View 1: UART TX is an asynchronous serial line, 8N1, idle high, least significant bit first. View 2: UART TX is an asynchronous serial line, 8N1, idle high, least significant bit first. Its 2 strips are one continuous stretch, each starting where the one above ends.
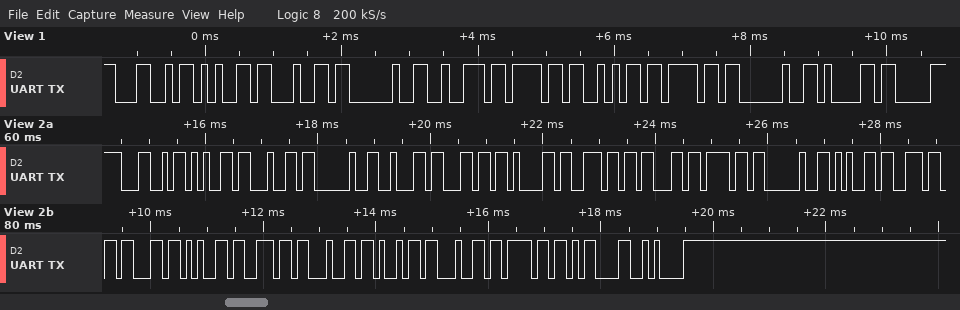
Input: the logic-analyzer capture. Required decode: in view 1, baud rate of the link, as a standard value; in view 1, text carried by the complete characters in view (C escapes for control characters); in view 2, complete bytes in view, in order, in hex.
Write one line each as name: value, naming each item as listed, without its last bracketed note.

in view 1, baud rate of the link, as a standard value: 9600 baud
in view 1, text carried by the complete characters in view: "Led rojo a"
in view 2, complete bytes in view, in order, in hex: 4C 65 64 20 62 6C 61 6E 63 6F 20 65 6E 63 65 6E 64 69 64 6F 0D 0A
